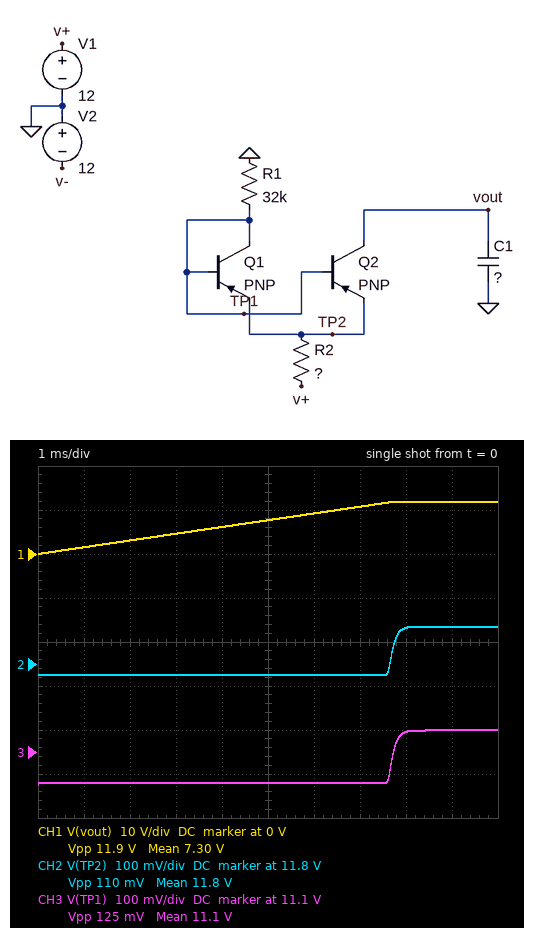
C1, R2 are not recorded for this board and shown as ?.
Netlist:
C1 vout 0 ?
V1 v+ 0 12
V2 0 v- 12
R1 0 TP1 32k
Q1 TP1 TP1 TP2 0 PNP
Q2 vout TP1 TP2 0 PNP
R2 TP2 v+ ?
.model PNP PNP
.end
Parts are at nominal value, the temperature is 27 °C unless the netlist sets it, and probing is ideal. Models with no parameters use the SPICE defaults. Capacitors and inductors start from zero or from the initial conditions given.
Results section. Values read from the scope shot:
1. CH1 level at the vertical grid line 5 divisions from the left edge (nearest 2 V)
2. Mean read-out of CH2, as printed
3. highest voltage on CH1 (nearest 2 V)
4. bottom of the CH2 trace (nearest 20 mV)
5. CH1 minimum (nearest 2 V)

8 V
11.8 V
12 V
11.78 V
0 V
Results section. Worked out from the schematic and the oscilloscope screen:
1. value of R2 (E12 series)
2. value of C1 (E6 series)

330 Ω
220 nF
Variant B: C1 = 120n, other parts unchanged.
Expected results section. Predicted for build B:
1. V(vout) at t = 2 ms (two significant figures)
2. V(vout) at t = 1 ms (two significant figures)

5.6 V
2.8 V
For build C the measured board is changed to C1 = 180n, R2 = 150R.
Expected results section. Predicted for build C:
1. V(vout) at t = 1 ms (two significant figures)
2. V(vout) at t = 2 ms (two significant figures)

1.9 V
3.8 V
